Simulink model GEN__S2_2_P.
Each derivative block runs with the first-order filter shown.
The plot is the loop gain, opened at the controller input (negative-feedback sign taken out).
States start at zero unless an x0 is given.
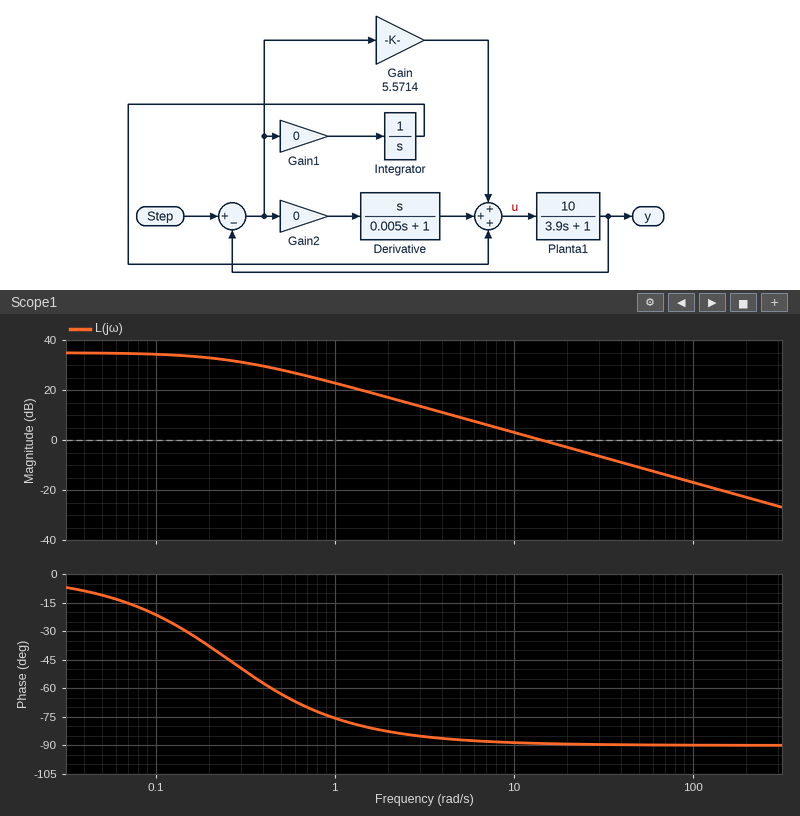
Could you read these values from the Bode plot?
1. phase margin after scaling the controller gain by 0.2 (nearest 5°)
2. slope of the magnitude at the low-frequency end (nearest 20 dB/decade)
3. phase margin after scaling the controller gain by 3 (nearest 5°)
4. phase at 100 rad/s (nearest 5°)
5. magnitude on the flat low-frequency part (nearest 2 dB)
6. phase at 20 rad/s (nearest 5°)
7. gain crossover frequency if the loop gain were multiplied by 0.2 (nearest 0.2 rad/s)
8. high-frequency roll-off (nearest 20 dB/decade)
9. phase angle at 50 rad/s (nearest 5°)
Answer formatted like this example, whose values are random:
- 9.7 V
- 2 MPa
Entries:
- 95°
- 0 dB/decade
- 90°
- -90°
- 34 dB
- -90°
- 2.8 rad/s
- -20 dB/decade
- -90°
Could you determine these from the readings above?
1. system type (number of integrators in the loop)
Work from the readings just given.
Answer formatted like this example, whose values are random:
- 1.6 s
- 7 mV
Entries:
- 0
